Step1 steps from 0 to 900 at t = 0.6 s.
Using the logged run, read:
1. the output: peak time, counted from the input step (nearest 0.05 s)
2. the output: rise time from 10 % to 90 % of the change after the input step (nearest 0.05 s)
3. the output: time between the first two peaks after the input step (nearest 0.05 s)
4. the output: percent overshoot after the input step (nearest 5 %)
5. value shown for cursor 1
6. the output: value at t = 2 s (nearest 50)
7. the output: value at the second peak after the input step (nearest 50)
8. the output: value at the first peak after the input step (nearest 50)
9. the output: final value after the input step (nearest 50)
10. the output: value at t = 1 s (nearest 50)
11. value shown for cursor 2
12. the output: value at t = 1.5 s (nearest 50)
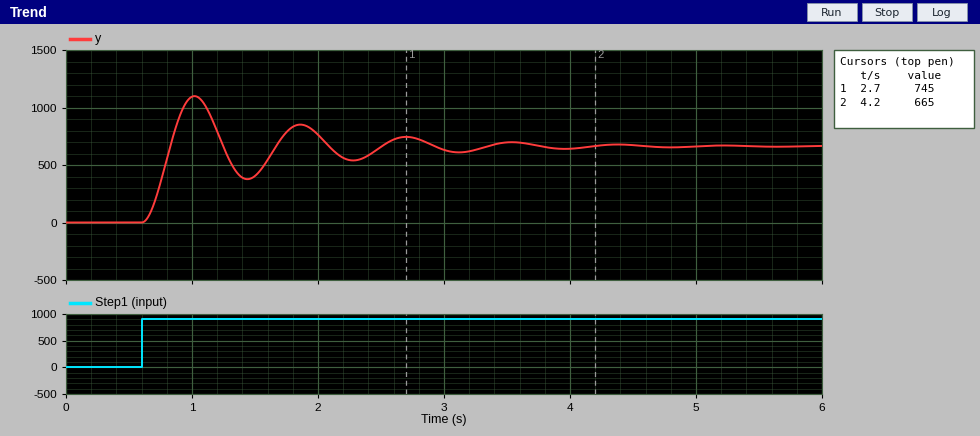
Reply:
0.40 s
0.15 s
0.85 s
65 %
745
750
850
1100
650
1100
665
400
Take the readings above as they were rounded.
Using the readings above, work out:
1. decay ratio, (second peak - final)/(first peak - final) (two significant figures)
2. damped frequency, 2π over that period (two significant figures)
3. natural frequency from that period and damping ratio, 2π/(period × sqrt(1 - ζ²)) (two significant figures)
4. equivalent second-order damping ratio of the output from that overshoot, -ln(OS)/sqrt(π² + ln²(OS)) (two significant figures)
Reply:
0.44
7.4 rad/s
7.5 rad/s
0.14
